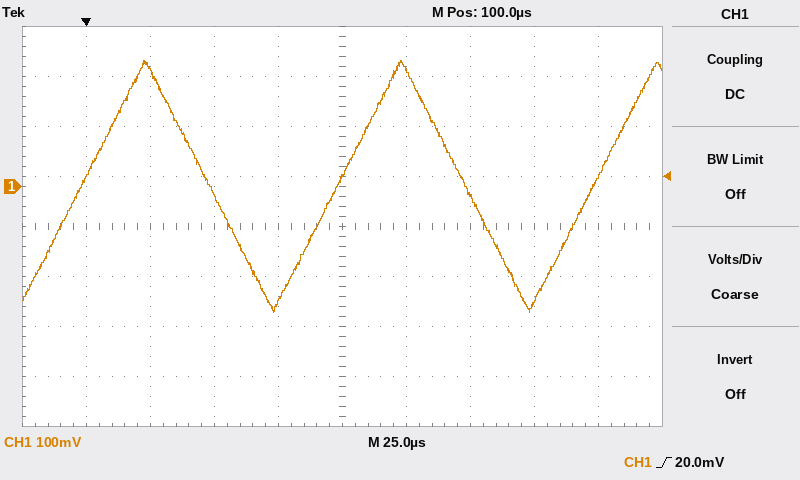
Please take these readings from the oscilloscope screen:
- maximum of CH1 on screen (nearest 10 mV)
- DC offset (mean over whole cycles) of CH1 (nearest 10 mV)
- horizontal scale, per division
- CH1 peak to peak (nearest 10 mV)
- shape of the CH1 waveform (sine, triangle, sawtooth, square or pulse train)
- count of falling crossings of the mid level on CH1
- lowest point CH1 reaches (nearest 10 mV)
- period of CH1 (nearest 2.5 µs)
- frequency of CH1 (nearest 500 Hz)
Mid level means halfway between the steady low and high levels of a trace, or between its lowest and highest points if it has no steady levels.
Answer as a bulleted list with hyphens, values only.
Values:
- 250 mV
- 0 mV
- 25 µs
- 500 mV
- triangle
- 2
- -250 mV
- 100.0 µs
- 10.0 kHz
